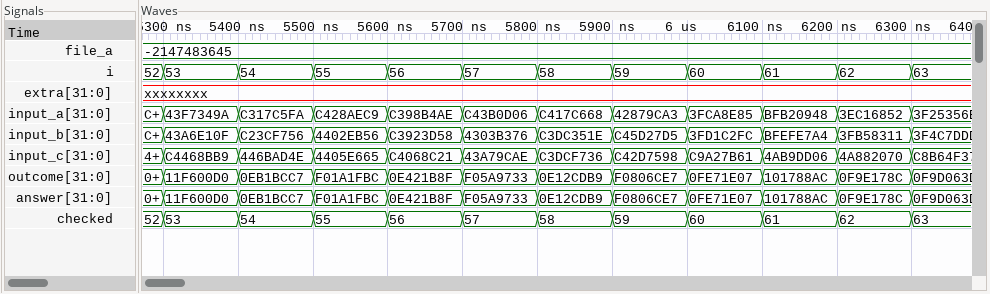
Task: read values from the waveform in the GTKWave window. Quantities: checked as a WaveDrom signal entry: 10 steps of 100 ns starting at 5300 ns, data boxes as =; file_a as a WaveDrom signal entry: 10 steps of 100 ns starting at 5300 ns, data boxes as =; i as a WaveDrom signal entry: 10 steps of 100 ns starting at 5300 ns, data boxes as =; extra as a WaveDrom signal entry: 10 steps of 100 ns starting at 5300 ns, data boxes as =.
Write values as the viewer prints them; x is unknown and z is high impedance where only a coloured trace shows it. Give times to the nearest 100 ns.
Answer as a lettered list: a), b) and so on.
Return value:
a) {name: 'checked', wave: '==========', data: '53 54 55 56 57 58 59 60 61 62'}
b) {name: 'file_a', wave: '=.........', data: '-2147483645'}
c) {name: 'i', wave: '==========', data: '53 54 55 56 57 58 59 60 61 62'}
d) {name: 'extra', wave: 'x.........'}
